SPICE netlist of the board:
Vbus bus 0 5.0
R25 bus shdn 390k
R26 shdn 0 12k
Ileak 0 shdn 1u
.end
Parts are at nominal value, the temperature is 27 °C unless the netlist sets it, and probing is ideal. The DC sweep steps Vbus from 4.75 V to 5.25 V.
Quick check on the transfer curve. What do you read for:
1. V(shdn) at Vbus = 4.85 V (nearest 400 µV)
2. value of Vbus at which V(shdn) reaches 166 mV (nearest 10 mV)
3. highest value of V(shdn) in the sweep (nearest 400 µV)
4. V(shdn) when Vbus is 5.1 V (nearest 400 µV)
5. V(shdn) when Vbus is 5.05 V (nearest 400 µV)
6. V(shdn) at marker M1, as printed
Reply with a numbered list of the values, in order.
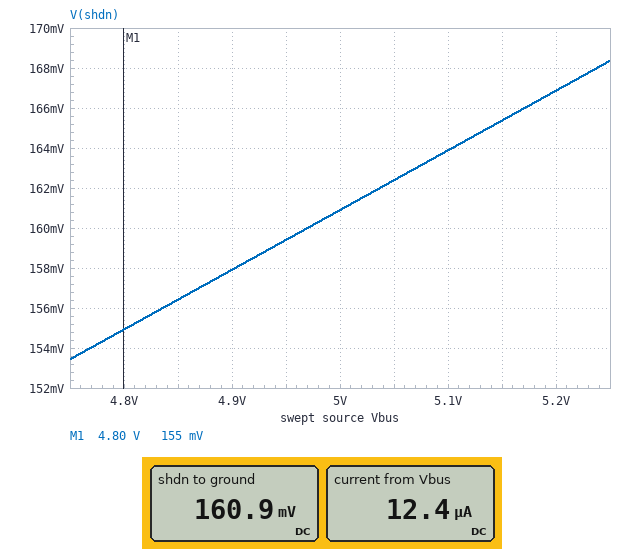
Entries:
1. 156.4 mV
2. 5.17 V
3. 168.4 mV
4. 164.0 mV
5. 162.4 mV
6. 155 mV
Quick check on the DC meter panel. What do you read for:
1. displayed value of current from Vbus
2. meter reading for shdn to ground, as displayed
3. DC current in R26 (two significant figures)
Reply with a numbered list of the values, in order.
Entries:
1. 12.4 µA
2. 160.9 mV
3. 13 µA
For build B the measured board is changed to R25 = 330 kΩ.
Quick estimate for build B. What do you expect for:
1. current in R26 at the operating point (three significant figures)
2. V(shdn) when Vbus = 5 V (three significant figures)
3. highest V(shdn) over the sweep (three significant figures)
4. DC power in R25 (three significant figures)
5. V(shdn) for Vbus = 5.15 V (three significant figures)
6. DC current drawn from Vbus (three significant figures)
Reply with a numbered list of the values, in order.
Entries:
1. 15.6 µA
2. 187 mV
3. 196 mV
4. 70.2 µW
5. 192 mV
6. 14.6 µA
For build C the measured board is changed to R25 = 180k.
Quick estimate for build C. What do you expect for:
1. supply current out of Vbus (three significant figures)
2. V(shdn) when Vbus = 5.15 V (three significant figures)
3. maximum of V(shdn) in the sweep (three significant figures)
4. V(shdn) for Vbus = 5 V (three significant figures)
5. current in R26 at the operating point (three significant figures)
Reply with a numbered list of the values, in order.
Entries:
1. 26.0 µA
2. 333 mV
3. 339 mV
4. 324 mV
5. 27.0 µA
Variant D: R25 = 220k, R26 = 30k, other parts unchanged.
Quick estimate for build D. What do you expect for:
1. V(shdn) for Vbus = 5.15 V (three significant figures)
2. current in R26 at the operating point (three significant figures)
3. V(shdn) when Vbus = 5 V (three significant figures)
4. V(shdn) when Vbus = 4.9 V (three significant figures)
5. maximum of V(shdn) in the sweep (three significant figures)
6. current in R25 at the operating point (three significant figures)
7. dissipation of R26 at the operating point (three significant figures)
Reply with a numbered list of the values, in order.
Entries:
1. 644 mV
2. 20.9 µA
3. 626 mV
4. 614 mV
5. 656 mV
6. 19.9 µA
7. 13.1 µW
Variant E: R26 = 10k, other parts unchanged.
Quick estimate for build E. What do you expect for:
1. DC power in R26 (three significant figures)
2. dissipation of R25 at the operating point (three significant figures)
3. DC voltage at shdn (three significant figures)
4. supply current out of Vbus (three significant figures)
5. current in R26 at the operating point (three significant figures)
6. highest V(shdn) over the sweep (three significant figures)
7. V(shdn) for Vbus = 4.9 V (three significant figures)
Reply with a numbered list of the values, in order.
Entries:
1. 1.82 µW
2. 60.7 µW
3. 135 mV
4. 12.5 µA
5. 13.5 µA
6. 141 mV
7. 132 mV
